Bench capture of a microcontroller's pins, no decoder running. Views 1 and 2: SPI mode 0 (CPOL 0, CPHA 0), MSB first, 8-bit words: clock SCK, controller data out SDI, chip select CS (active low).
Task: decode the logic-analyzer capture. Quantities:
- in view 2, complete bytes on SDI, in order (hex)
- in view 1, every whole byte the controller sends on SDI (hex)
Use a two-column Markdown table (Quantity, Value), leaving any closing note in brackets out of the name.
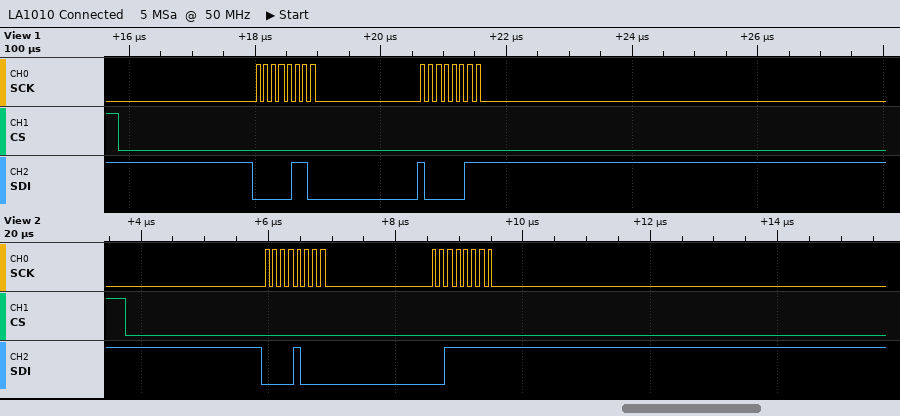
| Quantity | Value |
|---|---|
| in view 2, complete bytes on SDI, in order | 08 3F |
| in view 1, every whole byte the controller sends on SDI | 06 83 |
